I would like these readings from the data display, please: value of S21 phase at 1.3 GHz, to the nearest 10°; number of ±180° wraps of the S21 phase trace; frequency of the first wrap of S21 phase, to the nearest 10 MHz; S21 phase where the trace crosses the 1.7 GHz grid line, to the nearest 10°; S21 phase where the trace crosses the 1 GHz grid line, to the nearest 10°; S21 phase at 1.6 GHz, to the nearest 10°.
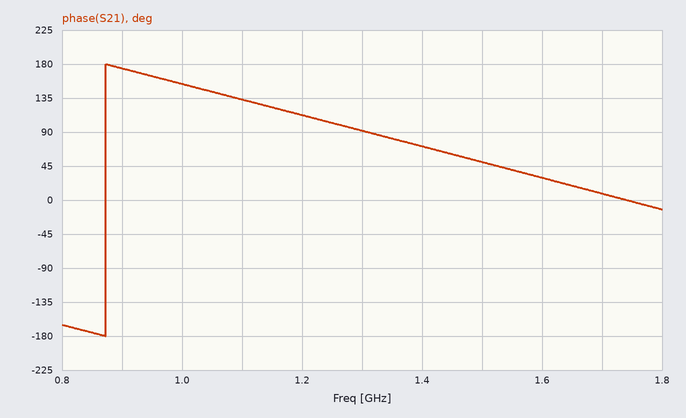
90°
1
870 MHz
10°
150°
30°
